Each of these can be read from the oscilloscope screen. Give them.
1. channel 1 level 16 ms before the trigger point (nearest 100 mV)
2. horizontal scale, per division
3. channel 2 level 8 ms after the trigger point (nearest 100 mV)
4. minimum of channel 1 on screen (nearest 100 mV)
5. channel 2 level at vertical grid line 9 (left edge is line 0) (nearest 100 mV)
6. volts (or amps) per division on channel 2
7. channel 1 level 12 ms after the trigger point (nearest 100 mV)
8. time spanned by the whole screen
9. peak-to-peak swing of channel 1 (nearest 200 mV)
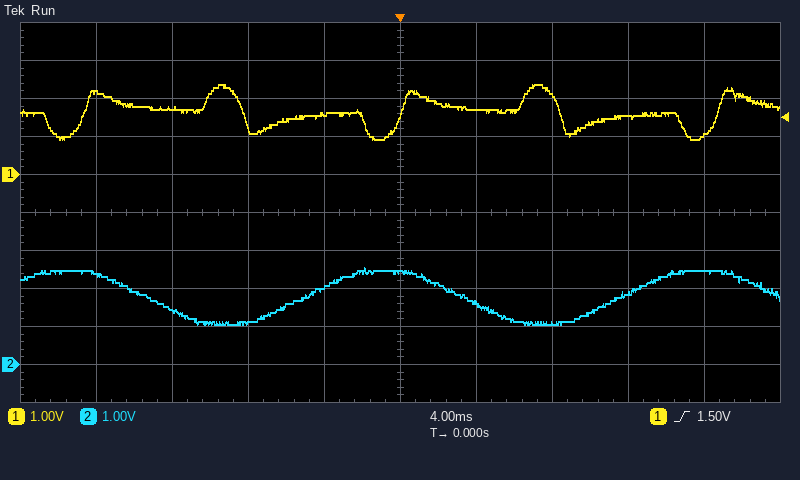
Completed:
2.2 V
4 ms
1.1 V
900 mV
2.5 V
1 V
1.5 V
40 ms
1.4 V
